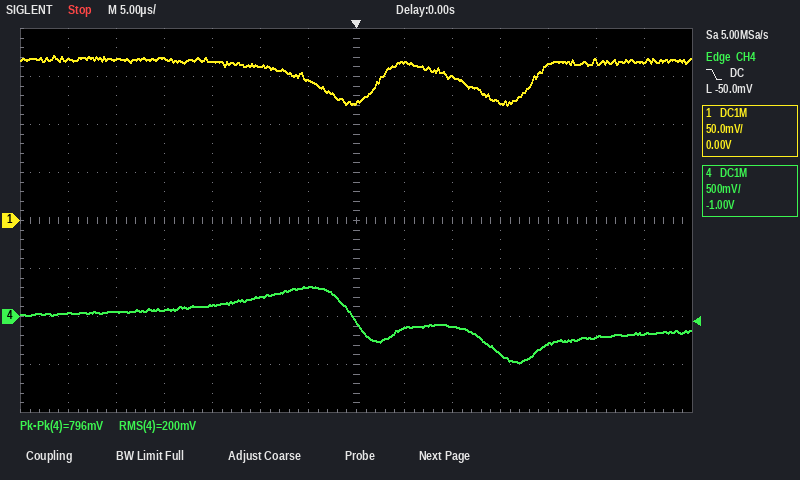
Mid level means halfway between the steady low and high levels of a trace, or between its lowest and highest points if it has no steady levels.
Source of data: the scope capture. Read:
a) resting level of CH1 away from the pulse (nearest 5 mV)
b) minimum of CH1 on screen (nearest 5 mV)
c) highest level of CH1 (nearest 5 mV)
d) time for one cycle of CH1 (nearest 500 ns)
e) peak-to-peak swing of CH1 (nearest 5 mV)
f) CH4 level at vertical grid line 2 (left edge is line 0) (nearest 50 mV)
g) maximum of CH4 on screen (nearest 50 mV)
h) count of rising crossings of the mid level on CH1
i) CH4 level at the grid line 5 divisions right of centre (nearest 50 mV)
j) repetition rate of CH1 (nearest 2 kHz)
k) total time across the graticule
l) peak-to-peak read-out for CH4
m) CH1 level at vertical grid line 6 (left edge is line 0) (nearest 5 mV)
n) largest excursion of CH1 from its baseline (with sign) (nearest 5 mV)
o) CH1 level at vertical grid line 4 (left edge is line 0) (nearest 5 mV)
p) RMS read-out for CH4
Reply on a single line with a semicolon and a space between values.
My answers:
165 mV; 120 mV; 170 mV; 16.0 µs; 50 mV; 50 mV; 300 mV; 2; -200 mV; 62 kHz; 70 µs; 796 mV; 145 mV; -45 mV; 165 mV; 200 mV
